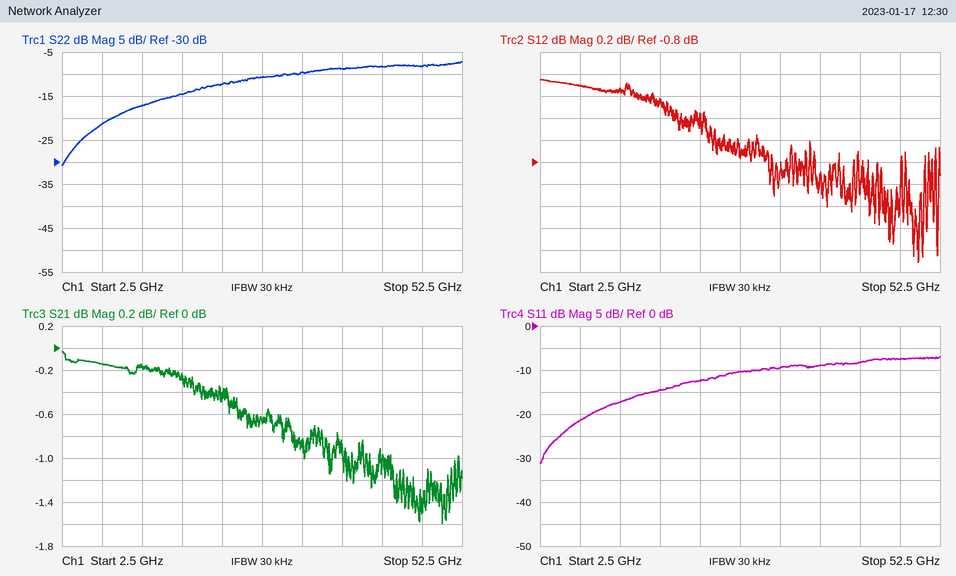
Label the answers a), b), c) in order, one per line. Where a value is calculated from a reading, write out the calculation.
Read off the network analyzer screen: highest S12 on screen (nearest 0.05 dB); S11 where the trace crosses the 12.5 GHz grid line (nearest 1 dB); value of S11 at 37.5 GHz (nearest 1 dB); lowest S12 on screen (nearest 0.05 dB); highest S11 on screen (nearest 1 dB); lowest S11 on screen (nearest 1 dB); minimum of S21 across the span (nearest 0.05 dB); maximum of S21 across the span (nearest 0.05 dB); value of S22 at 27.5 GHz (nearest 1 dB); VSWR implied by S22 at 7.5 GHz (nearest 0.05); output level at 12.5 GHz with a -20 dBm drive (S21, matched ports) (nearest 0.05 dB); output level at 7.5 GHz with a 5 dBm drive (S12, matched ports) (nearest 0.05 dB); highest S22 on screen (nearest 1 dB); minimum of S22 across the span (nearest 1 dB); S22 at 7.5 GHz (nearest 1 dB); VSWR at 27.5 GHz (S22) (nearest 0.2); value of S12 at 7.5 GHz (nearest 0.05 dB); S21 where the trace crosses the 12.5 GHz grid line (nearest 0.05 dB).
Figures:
a) -0.05 dB
b) -17 dB
c) -9 dB
d) -1.70 dB
e) -7 dB
f) -31 dB
g) -1.60 dB
h) -0.05 dB
i) -11 dB
j) |Γ| = 10^(-21/20) = 0.0891; VSWR = (1 + 0.0891)/(1 − 0.0891) ≈ 1.20
k) -20 dBm + (-0.15 dB) = -20.15 dBm
l) 5 dBm + (-0.10 dB) = 4.90 dBm
m) -7 dB
n) -31 dB
o) -21 dB
p) |Γ| = 10^(-11/20) = 0.2818; VSWR = (1 + 0.2818)/(1 − 0.2818) ≈ 1.8
q) -0.10 dB
r) -0.15 dB
